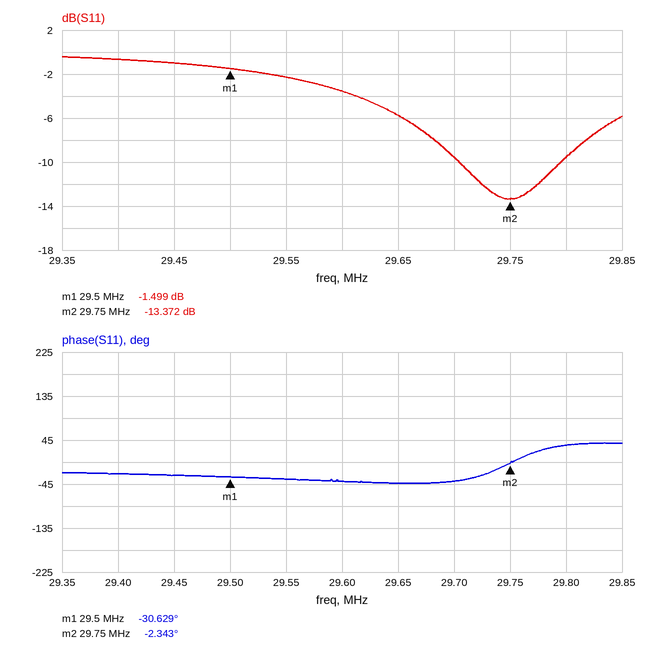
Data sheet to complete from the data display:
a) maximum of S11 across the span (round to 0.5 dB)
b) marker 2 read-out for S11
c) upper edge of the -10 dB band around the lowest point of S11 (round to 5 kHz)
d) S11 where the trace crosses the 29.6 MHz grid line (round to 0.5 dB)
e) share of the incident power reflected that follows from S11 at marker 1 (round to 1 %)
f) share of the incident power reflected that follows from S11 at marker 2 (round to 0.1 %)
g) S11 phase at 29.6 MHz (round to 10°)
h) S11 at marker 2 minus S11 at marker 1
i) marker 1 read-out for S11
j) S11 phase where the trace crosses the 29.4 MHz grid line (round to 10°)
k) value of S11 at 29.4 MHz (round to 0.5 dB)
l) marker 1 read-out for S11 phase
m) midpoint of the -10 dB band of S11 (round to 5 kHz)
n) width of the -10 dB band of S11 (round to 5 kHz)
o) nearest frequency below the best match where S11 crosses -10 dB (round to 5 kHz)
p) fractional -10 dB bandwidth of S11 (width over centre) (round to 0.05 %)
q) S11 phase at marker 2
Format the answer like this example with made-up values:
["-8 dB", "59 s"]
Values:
["-0.5 dB", "-13.372 dB", "29.795 MHz", "-3.5 dB", "71 %", "4.6 %", "-40°", "-11.873 dB", "-1.499 dB", "-20°", "-0.5 dB", "-30.629°", "29.750 MHz", "90 kHz", "29.705 MHz", "0.30 %", "-2.343°"]
